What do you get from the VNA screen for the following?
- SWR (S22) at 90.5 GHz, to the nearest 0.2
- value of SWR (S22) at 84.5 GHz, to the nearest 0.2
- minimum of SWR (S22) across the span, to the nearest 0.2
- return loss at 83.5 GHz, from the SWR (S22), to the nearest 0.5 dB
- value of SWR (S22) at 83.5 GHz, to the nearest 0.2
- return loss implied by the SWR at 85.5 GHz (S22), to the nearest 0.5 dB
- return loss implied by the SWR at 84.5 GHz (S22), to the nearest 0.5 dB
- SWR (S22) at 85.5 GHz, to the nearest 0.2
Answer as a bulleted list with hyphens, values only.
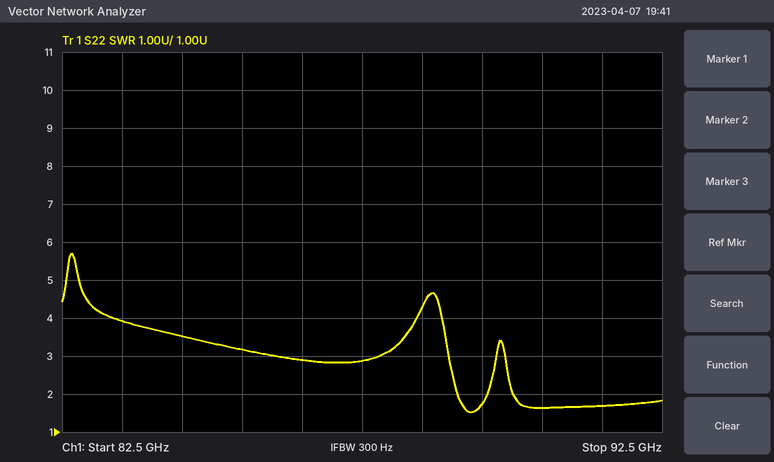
- 1.6
- 3.6
- 1.6
- 4.5 dB
- 4.0
- 5.5 dB
- 5.0 dB
- 3.2
